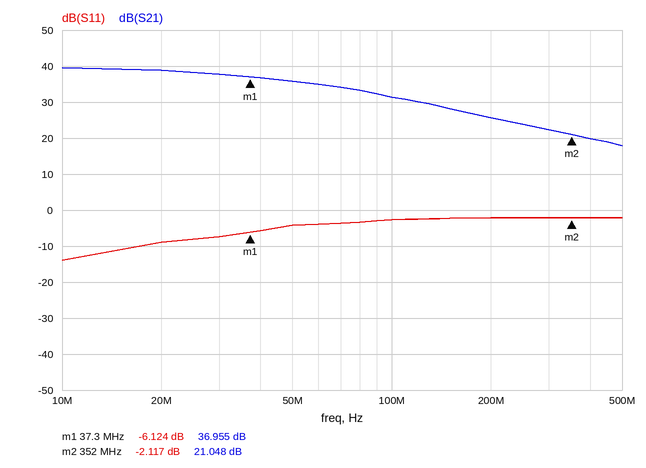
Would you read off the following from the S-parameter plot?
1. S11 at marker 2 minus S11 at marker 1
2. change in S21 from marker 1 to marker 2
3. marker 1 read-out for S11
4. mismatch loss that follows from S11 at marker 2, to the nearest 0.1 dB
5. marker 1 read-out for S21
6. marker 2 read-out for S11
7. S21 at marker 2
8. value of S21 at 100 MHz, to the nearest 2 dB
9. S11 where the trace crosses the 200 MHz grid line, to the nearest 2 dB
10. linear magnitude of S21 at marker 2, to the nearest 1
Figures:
4.007 dB
-15.907 dB
-6.124 dB
4.1 dB
36.955 dB
-2.117 dB
21.048 dB
32 dB
-2 dB
11
